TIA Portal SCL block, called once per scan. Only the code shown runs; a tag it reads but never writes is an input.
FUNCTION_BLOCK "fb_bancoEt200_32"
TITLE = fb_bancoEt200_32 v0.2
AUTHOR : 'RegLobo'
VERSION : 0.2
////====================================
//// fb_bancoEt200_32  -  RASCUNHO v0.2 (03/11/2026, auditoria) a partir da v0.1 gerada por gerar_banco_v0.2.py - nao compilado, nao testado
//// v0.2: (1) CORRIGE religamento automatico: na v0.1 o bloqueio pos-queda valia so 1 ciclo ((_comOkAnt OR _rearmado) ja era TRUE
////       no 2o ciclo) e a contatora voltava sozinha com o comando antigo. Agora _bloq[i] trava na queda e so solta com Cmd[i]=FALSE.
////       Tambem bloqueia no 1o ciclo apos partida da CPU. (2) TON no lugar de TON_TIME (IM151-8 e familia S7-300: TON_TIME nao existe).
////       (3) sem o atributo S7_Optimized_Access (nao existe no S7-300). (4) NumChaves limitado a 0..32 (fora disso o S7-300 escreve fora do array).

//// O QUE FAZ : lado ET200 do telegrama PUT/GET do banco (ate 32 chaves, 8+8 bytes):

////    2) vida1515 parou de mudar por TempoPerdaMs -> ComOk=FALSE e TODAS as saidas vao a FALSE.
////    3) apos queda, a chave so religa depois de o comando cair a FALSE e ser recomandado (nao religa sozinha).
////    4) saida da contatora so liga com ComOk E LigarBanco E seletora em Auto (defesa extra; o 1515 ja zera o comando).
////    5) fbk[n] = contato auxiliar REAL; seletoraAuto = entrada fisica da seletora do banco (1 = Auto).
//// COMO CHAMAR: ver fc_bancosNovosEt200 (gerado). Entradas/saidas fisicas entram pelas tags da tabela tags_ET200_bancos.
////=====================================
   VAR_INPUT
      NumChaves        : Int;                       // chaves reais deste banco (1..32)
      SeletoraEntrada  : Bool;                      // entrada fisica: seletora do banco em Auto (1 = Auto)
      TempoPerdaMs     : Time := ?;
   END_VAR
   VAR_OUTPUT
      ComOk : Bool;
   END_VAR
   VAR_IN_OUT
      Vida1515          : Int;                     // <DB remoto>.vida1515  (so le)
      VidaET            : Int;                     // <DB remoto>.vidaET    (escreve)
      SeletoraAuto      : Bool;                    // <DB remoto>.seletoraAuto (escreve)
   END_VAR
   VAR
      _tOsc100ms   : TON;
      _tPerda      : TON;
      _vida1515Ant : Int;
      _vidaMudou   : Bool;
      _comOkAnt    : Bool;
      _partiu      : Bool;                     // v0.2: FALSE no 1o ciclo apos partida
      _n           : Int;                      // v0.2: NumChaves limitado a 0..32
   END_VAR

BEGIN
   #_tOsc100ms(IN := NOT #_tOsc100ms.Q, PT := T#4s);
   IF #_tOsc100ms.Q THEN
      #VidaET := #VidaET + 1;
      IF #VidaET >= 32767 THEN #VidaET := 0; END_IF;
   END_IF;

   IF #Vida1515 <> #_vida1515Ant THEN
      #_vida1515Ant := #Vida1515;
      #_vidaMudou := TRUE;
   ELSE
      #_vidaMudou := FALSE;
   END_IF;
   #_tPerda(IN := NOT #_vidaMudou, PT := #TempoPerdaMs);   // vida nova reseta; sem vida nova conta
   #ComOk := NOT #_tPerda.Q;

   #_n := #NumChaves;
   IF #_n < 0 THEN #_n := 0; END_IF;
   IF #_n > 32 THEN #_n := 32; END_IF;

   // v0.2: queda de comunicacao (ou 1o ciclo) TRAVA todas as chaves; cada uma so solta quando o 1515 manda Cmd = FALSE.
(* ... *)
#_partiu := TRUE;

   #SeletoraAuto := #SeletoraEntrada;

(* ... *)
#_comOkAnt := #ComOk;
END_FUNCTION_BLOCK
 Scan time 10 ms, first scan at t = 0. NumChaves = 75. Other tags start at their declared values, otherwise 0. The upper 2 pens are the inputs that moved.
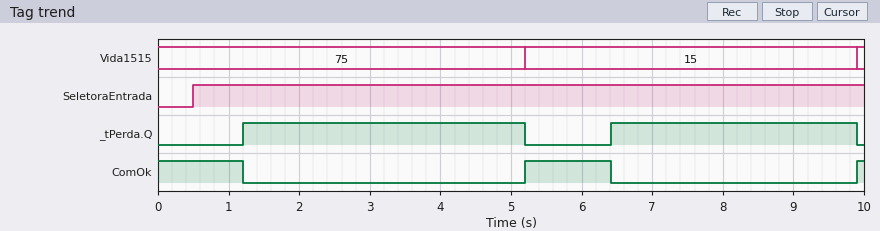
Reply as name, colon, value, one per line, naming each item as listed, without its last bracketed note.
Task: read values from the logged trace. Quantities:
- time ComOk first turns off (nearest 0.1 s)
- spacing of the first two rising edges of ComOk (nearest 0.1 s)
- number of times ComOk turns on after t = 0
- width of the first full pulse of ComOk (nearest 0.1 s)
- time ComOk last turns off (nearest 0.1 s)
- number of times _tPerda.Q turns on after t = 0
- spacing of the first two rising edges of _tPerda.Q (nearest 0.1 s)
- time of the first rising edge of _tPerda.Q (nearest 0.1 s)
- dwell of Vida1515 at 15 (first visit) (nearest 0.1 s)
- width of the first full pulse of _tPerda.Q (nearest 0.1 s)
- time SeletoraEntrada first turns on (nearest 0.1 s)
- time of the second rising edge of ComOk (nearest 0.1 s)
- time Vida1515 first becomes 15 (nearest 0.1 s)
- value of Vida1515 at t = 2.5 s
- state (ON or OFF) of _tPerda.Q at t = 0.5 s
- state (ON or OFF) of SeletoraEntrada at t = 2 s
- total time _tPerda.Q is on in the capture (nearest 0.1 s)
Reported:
time ComOk first turns off: 1.2 s
spacing of the first two rising edges of ComOk: 4.7 s
number of times ComOk turns on after t = 0: 2
width of the first full pulse of ComOk: 1.2 s
time ComOk last turns off: 6.4 s
number of times _tPerda.Q turns on after t = 0: 2
spacing of the first two rising edges of _tPerda.Q: 5.2 s
time of the first rising edge of _tPerda.Q: 1.2 s
dwell of Vida1515 at 15 (first visit): 4.7 s
width of the first full pulse of _tPerda.Q: 4.0 s
time SeletoraEntrada first turns on: 0.5 s
time of the second rising edge of ComOk: 9.9 s
time Vida1515 first becomes 15: 5.2 s
value of Vida1515 at t = 2.5 s: 75
state (ON or OFF) of _tPerda.Q at t = 0.5 s: OFF
state (ON or OFF) of SeletoraEntrada at t = 2 s: ON
total time _tPerda.Q is on in the capture: 7.5 s
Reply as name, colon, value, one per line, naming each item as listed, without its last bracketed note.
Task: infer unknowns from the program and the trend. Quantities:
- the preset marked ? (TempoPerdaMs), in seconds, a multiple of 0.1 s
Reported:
the preset marked ? (TempoPerdaMs), in seconds, a multiple of 0.1 s: 1.2 s
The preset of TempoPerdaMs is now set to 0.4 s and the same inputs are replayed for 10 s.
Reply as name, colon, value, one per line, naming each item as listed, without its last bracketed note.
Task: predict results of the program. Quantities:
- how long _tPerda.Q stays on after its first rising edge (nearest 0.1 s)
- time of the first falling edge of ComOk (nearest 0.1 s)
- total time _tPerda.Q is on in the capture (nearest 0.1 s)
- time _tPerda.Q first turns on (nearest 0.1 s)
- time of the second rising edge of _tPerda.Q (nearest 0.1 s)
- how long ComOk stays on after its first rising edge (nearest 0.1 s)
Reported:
how long _tPerda.Q stays on after its first rising edge: 4.8 s
time of the first falling edge of ComOk: 0.4 s
total time _tPerda.Q is on in the capture: 9.1 s
time _tPerda.Q first turns on: 0.4 s
time of the second rising edge of _tPerda.Q: 5.6 s
how long ComOk stays on after its first rising edge: 0.4 s
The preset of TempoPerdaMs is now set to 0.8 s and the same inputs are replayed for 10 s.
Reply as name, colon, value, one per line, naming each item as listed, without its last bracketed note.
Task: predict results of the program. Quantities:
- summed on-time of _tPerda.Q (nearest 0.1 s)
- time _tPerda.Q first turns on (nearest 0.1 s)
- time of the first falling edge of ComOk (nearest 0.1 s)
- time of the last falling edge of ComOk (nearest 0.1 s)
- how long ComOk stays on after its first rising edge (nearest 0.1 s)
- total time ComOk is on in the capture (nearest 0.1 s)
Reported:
summed on-time of _tPerda.Q: 8.3 s
time _tPerda.Q first turns on: 0.8 s
time of the first falling edge of ComOk: 0.8 s
time of the last falling edge of ComOk: 6.0 s
how long ComOk stays on after its first rising edge: 0.8 s
total time ComOk is on in the capture: 1.7 s
